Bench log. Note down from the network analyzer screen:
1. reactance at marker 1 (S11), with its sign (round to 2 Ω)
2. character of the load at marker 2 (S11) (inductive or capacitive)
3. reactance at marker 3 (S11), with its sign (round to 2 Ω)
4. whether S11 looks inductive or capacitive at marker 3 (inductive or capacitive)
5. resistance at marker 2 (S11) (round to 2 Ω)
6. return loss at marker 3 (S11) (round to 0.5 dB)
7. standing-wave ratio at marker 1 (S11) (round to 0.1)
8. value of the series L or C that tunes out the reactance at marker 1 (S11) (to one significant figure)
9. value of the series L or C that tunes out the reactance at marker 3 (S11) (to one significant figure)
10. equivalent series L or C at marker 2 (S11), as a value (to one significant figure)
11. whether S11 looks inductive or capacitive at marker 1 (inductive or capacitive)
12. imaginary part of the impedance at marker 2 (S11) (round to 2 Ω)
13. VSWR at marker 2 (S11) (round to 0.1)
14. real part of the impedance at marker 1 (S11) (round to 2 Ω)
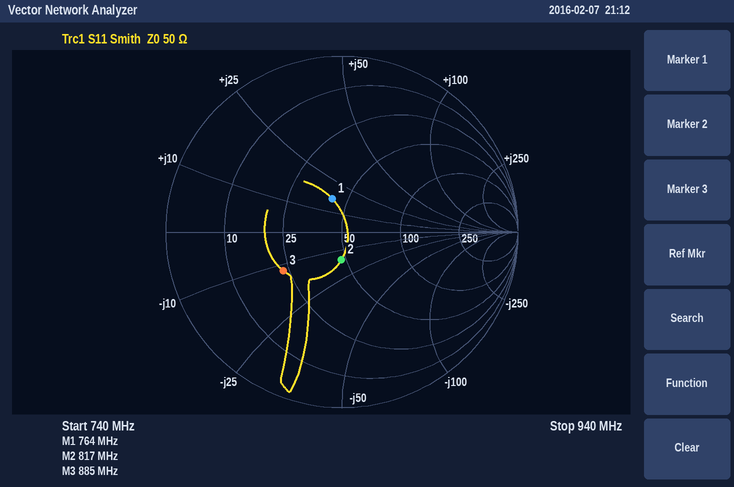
+16 Ω
capacitive
-12 Ω
capacitive
48 Ω
8.0 dB
1.5
10 pF
2 nH
10 pF
inductive
-16 Ω
1.4
42 Ω
